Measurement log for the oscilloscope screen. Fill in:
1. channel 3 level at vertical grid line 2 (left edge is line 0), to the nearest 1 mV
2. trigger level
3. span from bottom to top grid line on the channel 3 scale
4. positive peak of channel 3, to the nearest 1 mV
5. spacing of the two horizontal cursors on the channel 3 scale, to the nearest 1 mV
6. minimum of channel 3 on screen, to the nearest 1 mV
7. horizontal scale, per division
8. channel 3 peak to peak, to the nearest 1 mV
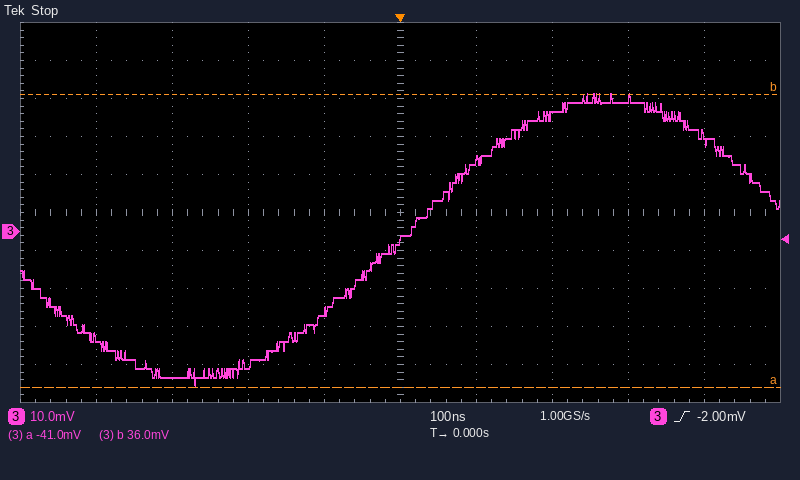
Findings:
-38 mV
-2.00 mV
100 mV
36 mV
77 mV
-41 mV
100 ns
77 mV
